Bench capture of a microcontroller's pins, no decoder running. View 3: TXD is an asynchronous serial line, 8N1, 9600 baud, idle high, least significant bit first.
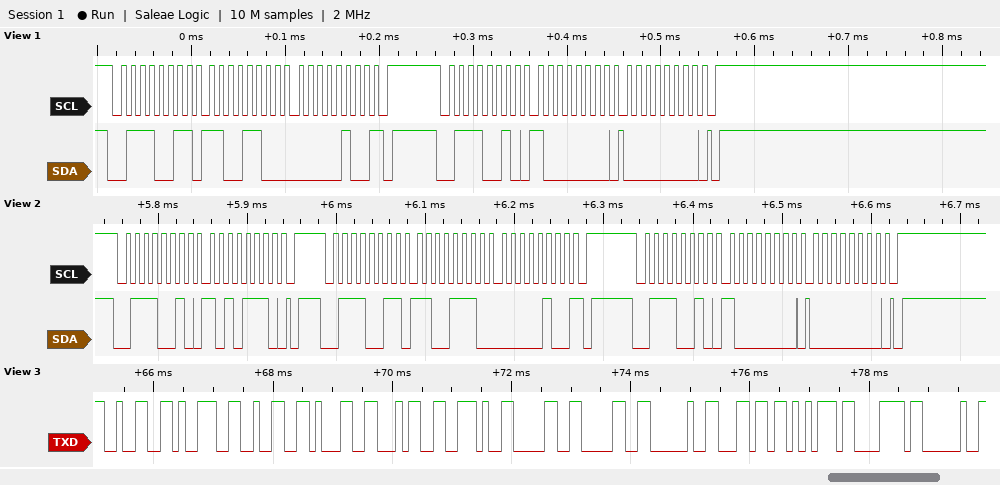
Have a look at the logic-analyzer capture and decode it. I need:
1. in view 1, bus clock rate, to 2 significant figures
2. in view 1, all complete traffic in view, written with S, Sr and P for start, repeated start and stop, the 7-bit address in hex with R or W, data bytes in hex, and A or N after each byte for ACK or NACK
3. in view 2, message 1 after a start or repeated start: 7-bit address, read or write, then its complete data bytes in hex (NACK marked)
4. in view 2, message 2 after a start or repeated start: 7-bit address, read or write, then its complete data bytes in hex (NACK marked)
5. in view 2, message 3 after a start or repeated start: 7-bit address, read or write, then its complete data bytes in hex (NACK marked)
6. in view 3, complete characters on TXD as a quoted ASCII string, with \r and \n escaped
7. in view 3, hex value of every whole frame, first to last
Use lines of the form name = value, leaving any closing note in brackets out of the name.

in view 1, bus clock rate, to 2 significant figures = 100 kHz
in view 1, all complete traffic in view, written with S, Sr and P for start, repeated start and stop, the 7-bit address in hex with R or W, data bytes in hex, and A or N after each byte for ACK or NACK = S 39R A CC A 04 N P S 39W A 80 A 00 A P
in view 2, message 1 after a start or repeated start: 7-bit address, read or write, then its complete data bytes in hex = 0x39 write: AE
in view 2, message 2 after a start or repeated start: 7-bit address, read or write, then its complete data bytes in hex = 0x39 read: CE 04 NACK
in view 2, message 3 after a start or repeated start: 7-bit address, read or write, then its complete data bytes in hex = 0x39 write: 80 00
in view 3, complete characters on TXD as a quoted ASCII string, with \r and \n escaped = "29214.00 lux "
in view 3, hex value of every whole frame, first to last = 32 39 32 31 34 2E 30 30 20 6C 75 78 20
